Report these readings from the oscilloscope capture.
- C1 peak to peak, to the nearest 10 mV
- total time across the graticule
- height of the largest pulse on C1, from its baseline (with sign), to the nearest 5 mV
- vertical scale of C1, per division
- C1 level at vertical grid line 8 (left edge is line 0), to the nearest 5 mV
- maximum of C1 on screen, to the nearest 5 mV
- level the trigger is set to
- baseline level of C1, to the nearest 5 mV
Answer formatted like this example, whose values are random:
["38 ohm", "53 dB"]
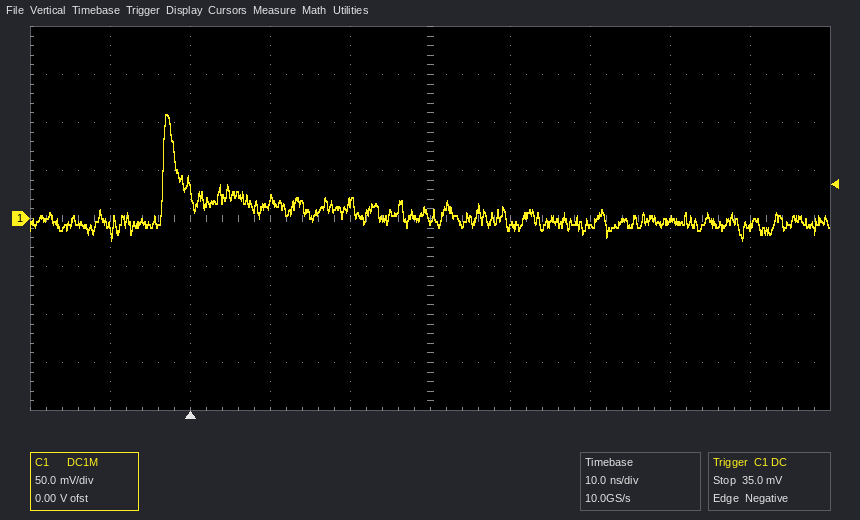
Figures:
["130 mV", "100 ns", "+110 mV", "50 mV", "0 mV", "110 mV", "35.0 mV", "0 mV"]
